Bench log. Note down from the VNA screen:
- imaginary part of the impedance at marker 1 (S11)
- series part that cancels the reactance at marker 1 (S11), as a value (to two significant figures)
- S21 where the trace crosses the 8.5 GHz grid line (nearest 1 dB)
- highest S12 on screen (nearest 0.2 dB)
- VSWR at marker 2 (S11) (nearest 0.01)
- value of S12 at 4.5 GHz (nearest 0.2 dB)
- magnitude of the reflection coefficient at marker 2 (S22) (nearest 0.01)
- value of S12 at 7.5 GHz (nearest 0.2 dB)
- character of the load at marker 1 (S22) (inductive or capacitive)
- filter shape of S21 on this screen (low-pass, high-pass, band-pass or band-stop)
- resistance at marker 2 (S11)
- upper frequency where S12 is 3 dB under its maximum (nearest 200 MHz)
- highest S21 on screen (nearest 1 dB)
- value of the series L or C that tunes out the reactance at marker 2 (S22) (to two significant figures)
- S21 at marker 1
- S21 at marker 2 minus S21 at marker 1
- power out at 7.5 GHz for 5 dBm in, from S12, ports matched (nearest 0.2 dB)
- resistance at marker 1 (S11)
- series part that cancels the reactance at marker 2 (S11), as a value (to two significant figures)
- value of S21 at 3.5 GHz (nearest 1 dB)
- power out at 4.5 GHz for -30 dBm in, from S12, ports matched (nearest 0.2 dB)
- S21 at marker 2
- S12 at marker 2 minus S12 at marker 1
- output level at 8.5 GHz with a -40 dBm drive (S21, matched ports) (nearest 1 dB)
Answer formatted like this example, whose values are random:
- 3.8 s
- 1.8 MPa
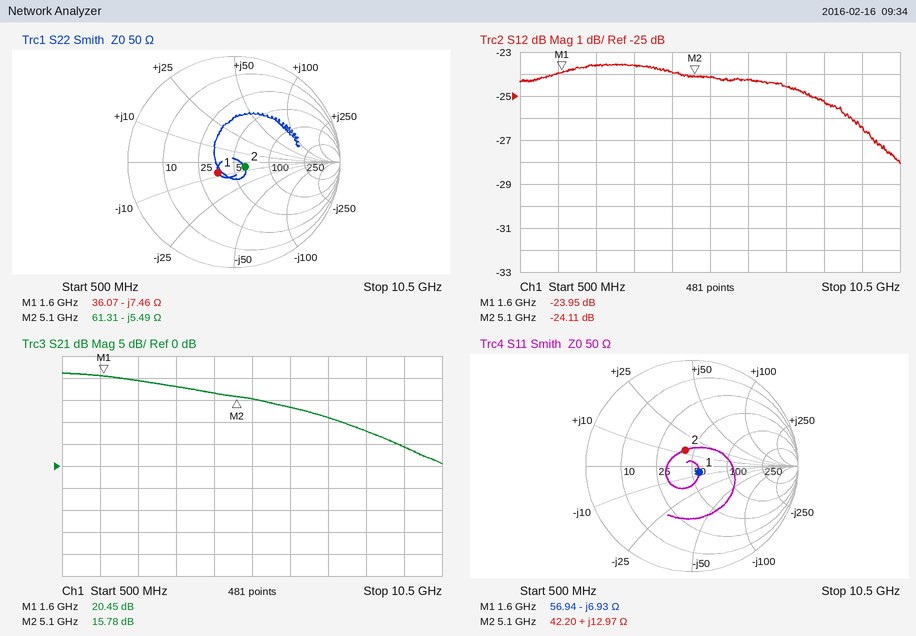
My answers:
- -6.93 Ω
- 690 pH
- 8 dB
- -23.6 dB
- 1.39
- -24.0 dB
- 0.11
- -24.6 dB
- capacitive
- low-pass
- 42.20 Ω
- 9.6 GHz
- 21 dB
- 170 pH
- 20.45 dB
- -4.67 dB
- -19.6 dBm
- 56.94 Ω
- 2.4 pF
- 18 dB
- -54.0 dBm
- 15.78 dB
- -0.16 dB
- -32 dBm
